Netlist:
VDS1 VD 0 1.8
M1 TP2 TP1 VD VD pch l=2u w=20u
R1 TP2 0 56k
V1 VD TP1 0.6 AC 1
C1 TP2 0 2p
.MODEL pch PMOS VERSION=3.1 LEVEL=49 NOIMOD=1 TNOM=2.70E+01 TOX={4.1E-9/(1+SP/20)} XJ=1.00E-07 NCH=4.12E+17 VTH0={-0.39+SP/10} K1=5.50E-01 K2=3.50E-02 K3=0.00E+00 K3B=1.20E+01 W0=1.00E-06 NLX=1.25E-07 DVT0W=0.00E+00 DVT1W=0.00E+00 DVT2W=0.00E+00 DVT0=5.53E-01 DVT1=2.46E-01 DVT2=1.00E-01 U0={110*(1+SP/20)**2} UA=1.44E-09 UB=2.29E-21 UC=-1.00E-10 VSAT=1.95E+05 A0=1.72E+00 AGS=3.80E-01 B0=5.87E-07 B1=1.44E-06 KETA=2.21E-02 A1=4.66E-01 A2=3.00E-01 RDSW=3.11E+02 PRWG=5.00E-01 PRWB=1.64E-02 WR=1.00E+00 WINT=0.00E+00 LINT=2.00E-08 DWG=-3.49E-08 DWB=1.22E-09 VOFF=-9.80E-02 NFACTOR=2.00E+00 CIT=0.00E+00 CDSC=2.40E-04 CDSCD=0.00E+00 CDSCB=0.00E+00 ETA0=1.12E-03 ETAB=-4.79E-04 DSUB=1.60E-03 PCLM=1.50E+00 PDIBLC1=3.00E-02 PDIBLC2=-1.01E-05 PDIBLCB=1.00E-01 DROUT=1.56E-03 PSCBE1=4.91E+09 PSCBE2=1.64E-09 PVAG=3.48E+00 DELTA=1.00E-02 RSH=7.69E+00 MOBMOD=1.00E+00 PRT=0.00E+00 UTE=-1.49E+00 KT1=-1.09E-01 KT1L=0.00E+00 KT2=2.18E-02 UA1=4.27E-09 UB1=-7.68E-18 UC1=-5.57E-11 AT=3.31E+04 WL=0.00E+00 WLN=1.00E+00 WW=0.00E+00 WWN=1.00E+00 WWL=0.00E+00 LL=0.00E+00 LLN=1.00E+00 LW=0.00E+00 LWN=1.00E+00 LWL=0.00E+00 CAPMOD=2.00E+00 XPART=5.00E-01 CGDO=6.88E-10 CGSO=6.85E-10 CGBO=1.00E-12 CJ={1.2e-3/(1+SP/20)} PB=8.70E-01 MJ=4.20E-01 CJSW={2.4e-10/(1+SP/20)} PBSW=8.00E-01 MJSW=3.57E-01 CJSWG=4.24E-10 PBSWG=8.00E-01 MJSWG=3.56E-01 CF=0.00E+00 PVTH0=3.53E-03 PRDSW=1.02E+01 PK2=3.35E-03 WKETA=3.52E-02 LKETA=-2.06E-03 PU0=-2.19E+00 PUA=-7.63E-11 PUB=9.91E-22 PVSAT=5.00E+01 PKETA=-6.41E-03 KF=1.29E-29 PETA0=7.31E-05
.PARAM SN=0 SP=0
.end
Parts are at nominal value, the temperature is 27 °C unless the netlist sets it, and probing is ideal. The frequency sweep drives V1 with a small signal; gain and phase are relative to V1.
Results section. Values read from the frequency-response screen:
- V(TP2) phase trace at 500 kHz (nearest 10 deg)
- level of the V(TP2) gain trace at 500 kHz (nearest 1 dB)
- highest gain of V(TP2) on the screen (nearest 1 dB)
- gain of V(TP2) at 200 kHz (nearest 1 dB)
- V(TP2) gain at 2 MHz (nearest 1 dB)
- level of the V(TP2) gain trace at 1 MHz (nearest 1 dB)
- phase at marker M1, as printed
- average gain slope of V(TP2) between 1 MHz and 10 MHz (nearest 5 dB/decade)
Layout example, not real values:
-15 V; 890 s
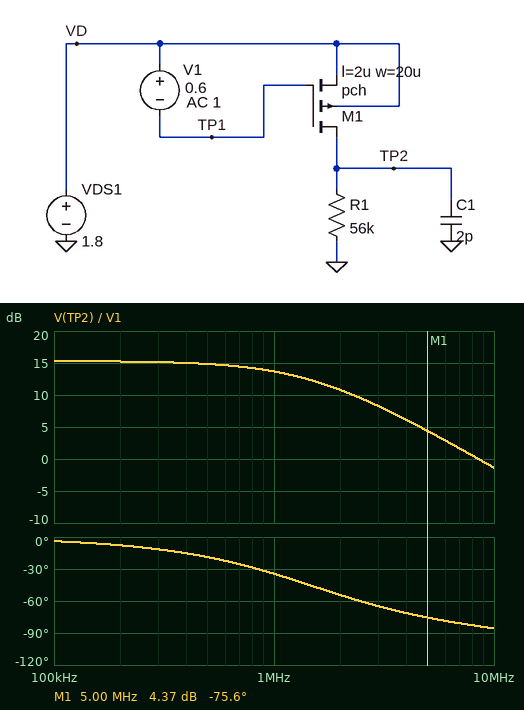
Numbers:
-20 deg; 15 dB; 15 dB; 15 dB; 11 dB; 14 dB; -75.6 deg; -15 dB/decade
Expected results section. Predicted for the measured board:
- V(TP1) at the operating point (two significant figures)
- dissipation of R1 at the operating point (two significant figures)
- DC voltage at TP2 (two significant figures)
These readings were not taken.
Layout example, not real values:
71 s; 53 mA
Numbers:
1.2 V; 7.5 µW; 650 mV
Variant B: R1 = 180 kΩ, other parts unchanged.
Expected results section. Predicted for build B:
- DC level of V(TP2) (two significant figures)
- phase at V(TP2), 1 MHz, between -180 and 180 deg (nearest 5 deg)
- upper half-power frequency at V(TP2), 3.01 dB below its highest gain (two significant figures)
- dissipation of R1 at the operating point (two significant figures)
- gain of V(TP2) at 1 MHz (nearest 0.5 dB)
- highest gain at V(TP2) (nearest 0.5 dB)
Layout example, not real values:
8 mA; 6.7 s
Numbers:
1.7 V; -20 deg; 2.9 MHz; 16 µW; 5.5 dB; 6.0 dB
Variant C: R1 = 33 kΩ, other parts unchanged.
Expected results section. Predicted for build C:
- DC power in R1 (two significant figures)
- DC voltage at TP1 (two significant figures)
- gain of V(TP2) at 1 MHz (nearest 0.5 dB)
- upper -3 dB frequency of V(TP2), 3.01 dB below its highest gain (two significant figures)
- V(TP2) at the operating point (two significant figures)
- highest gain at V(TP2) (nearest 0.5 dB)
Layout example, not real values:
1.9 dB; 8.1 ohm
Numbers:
4.6 µW; 1.2 V; 10.5 dB; 2.5 MHz; 390 mV; 11.0 dB
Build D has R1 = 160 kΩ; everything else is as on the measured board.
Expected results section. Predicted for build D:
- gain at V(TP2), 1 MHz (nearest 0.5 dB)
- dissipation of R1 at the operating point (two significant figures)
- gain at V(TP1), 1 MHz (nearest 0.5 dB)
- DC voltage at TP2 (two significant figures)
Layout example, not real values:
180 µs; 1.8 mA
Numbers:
12.0 dB; 17 µW; 0 dB; 1.6 V
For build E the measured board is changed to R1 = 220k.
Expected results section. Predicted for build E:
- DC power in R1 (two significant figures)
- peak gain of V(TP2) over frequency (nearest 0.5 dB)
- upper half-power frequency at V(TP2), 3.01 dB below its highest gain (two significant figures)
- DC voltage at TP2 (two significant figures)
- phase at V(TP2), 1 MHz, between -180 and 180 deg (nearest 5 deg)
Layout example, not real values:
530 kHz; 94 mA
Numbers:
13 µW; -0.5 dB; 4.6 MHz; 1.7 V; -15 deg
